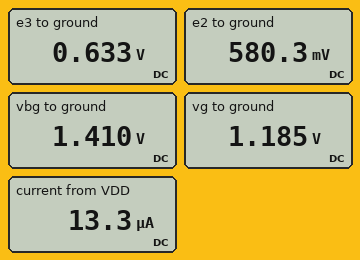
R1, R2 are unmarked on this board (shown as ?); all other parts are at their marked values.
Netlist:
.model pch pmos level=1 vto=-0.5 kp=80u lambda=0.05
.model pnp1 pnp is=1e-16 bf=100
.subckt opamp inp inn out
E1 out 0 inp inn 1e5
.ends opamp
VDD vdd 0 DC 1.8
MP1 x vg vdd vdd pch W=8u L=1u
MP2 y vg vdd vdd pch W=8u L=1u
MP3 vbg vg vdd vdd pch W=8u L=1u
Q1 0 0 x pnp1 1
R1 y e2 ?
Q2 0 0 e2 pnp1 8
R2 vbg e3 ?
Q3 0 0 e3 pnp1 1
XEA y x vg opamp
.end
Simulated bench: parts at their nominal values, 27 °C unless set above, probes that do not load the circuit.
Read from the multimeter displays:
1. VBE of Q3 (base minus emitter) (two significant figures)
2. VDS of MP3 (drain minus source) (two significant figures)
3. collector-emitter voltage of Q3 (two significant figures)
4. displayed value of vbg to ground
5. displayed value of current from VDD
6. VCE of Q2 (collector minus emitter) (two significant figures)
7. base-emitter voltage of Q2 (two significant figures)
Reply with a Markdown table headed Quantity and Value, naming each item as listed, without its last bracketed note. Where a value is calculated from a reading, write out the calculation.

| Quantity | Value |
|---|---|
| VBE of Q3 (base minus emitter) | 0 V - 633 mV = -630 mV |
| VDS of MP3 (drain minus source) | 1.41 V - 1.8 V = -390 mV |
| collector-emitter voltage of Q3 | 0 V - 633 mV = -630 mV |
| displayed value of vbg to ground | 1.410 V |
| displayed value of current from VDD | 13.3 µA |
| VCE of Q2 (collector minus emitter) | 0 V - 580.3 mV = -580 mV |
| base-emitter voltage of Q2 | 0 V - 580.3 mV = -580 mV |
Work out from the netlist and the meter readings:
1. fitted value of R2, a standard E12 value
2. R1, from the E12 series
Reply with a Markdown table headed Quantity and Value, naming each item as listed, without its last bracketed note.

| Quantity | Value |
|---|---|
| fitted value of R2, a standard E12 value | 180 kΩ |
| R1, from the E12 series | 12 kΩ |
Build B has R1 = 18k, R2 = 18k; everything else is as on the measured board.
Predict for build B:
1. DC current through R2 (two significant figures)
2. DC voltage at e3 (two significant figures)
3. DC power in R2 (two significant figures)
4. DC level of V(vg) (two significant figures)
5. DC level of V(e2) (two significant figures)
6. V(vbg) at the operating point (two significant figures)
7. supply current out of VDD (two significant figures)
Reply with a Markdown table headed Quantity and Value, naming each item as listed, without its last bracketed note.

| Quantity | Value |
|---|---|
| DC current through R2 | 3.0 µA |
| DC voltage at e3 | 620 mV |
| DC power in R2 | 160 nW |
| DC level of V(vg) | 1.2 V |
| DC level of V(e2) | 570 mV |
| V(vbg) at the operating point | 680 mV |
| supply current out of VDD | 9.0 µA |
